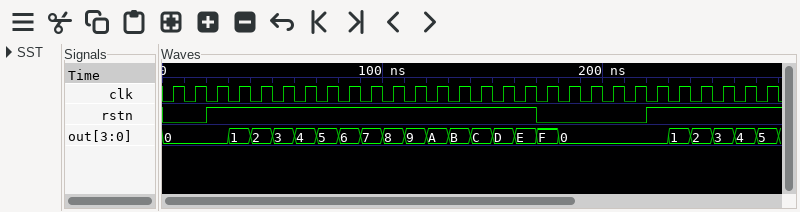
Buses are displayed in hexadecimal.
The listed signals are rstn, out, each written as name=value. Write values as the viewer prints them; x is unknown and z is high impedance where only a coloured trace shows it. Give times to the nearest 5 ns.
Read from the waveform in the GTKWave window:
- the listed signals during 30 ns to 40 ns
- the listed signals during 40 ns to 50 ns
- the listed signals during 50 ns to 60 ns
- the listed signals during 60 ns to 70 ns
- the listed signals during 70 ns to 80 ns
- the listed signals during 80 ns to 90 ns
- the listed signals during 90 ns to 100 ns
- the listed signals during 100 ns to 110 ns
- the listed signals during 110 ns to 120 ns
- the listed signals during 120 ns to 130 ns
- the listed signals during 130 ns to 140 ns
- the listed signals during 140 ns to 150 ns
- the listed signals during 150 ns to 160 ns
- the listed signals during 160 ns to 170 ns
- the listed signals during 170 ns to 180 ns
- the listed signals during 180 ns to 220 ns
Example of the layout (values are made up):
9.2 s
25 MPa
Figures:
rstn=1, out=1
rstn=1, out=2
rstn=1, out=3
rstn=1, out=4
rstn=1, out=5
rstn=1, out=6
rstn=1, out=7
rstn=1, out=8
rstn=1, out=9
rstn=1, out=A
rstn=1, out=B
rstn=1, out=C
rstn=1, out=D
rstn=1, out=E
rstn=0, out=F
rstn=0, out=0
